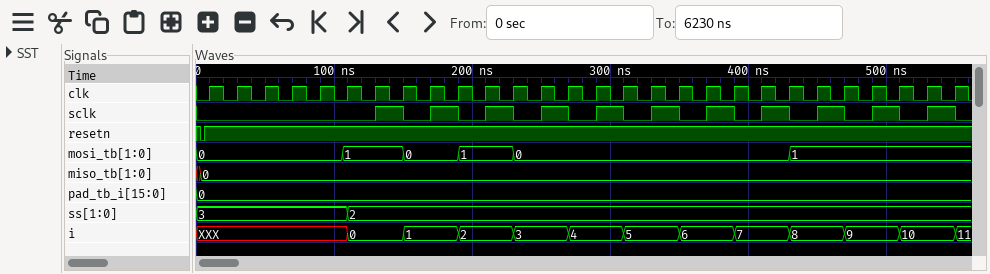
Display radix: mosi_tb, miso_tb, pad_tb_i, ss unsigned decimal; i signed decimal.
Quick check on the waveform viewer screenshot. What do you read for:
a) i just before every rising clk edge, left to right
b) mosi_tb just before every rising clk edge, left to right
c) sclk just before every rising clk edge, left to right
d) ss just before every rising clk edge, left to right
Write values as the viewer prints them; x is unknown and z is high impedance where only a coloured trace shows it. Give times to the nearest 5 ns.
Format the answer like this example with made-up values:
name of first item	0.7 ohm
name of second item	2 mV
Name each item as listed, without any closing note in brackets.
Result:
i just before every rising clk edge, left to right	XXX, XXX, XXX, XXX, XXX, XXX, 0, 0, 1, 1, 2, 2, 3, 3, 4, 4, 5, 5, 6, 6, 7, 7, 8, 8, 9, 9, 10, 10
mosi_tb just before every rising clk edge, left to right	0, 0, 0, 0, 0, 1, 1, 1, 0, 0, 1, 1, 0, 0, 0, 0, 0, 0, 0, 0, 0, 0, 1, 1, 1, 1, 1, 1
sclk just before every rising clk edge, left to right	0 0 0 0 0 0 0 1 0 1 0 1 0 1 0 1 0 1 0 1 0 1 0 1 0 1 0 1
ss just before every rising clk edge, left to right	3, 3, 3, 3, 3, 3, 2, 2, 2, 2, 2, 2, 2, 2, 2, 2, 2, 2, 2, 2, 2, 2, 2, 2, 2, 2, 2, 2
